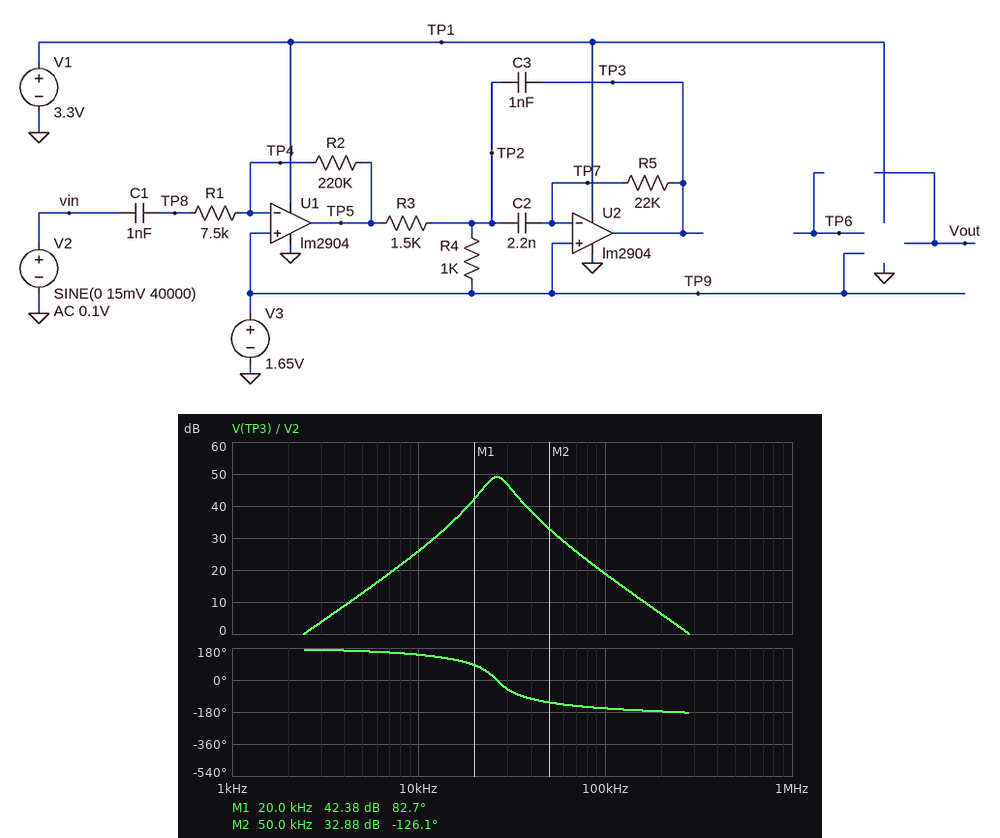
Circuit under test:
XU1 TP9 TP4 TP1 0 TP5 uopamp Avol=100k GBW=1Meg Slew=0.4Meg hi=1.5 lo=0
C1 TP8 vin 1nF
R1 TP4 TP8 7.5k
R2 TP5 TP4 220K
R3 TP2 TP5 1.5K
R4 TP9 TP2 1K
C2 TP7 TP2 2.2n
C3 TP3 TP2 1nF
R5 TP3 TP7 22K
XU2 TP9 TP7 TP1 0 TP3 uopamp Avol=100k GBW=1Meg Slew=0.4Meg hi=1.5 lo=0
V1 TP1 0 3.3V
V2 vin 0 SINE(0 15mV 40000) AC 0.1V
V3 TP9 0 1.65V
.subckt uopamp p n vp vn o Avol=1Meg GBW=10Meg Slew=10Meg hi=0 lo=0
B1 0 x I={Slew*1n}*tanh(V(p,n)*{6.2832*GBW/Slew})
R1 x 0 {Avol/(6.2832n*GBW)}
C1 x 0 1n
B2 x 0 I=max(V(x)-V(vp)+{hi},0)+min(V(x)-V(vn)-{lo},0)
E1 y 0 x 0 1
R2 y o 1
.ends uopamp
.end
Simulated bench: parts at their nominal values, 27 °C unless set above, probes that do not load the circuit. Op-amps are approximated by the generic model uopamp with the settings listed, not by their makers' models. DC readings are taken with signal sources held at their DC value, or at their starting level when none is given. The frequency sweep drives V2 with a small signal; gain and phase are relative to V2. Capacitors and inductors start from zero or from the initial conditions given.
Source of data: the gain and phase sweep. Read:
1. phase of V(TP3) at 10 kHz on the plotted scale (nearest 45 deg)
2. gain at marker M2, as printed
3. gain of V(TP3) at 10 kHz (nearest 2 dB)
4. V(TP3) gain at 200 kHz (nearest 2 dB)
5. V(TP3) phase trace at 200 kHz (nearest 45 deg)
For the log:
135 deg
32.88 dB
26 dB
6 dB
-180 deg
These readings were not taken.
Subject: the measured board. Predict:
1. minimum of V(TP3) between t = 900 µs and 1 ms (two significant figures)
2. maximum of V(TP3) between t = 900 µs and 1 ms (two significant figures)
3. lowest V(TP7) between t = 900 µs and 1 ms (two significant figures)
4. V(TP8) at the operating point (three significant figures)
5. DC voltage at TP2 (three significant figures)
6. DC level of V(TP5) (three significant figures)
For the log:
1.3 V
1.8 V
1.5 V
1.65 V
1.65 V
1.65 V
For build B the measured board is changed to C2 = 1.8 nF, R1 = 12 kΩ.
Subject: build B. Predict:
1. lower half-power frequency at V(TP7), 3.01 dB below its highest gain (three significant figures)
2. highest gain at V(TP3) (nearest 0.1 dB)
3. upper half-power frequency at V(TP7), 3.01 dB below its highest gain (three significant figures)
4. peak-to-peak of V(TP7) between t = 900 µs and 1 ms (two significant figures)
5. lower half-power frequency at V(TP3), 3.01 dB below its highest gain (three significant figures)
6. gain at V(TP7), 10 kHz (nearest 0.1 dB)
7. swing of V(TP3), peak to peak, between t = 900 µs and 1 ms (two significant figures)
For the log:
25.8 kHz
44.4 dB
35.5 kHz
130 mV
24.8 kHz
-17.4 dB
480 mV
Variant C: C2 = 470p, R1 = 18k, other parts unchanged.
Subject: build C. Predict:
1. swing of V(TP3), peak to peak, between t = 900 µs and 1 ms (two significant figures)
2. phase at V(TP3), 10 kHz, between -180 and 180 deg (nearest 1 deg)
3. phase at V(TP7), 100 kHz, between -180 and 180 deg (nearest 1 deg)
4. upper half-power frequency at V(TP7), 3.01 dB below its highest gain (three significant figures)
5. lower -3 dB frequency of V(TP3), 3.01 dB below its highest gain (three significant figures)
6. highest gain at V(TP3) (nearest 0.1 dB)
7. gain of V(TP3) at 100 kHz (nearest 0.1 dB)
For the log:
490 mV
123 deg
140 deg
69.0 kHz
47.3 kHz
33.5 dB
19.2 dB
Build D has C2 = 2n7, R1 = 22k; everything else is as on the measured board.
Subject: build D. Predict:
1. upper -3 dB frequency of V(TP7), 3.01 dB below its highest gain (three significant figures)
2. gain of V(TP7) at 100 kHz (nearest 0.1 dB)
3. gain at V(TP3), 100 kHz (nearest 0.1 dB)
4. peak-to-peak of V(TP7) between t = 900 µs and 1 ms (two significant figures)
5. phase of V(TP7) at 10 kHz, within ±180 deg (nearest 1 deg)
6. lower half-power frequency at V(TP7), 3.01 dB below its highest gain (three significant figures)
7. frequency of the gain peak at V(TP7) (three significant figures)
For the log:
30.2 kHz
-4.3 dB
15.7 dB
87 mV
21 deg
21.0 kHz
24.4 kHz
